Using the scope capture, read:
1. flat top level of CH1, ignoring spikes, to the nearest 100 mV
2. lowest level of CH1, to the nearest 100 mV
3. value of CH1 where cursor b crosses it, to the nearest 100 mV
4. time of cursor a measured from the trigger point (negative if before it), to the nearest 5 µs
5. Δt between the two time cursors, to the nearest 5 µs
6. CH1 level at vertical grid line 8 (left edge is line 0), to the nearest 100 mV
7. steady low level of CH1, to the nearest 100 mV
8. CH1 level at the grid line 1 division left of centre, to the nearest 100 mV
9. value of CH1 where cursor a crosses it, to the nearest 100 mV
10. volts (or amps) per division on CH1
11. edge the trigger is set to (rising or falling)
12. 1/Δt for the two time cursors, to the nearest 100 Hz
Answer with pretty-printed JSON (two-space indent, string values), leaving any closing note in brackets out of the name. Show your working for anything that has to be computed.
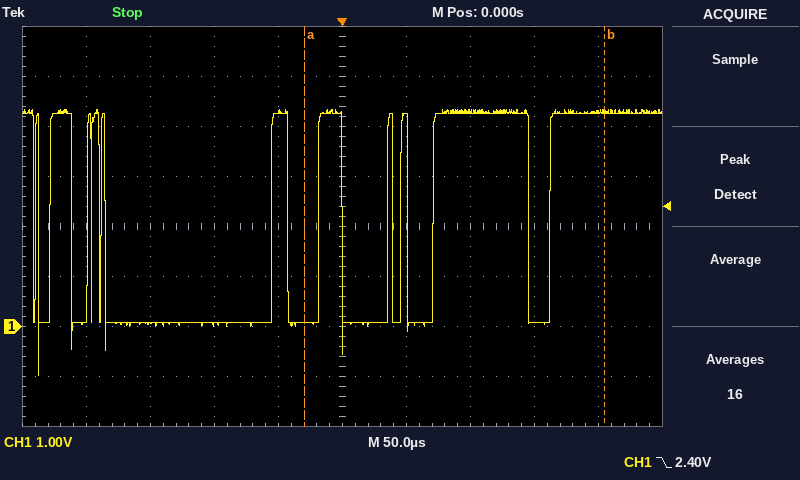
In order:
{
  "flat top level of CH1, ignoring spikes, to the nearest 100 mV": "4.3 V",
  "lowest level of CH1, to the nearest 100 mV": "-1.0 V",
  "value of CH1 where cursor b crosses it, to the nearest 100 mV": "4.3 V",
  "time of cursor a measured from the trigger point (negative if before it), to the nearest 5 µs": "-30 µs",
  "Δt between the two time cursors, to the nearest 5 µs": "235 µs",
  "CH1 level at vertical grid line 8 (left edge is line 0), to the nearest 100 mV": "100 mV",
  "steady low level of CH1, to the nearest 100 mV": "100 mV",
  "CH1 level at the grid line 1 division left of centre, to the nearest 100 mV": "4.3 V",
  "value of CH1 where cursor a crosses it, to the nearest 100 mV": "100 mV",
  "volts (or amps) per division on CH1": "1 V",
  "edge the trigger is set to": "falling",
  "1/Δt for the two time cursors, to the nearest 100 Hz": "1 / 235 µs ≈ 4.3 kHz"
}
